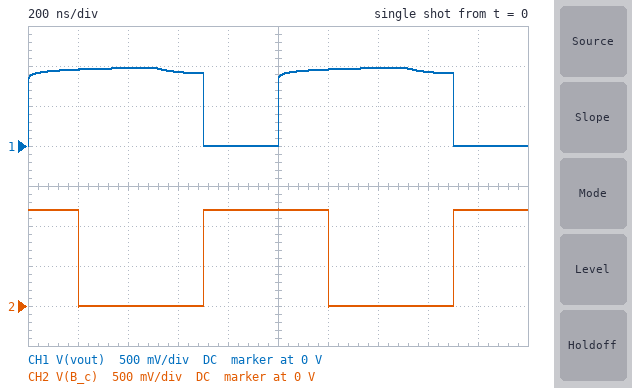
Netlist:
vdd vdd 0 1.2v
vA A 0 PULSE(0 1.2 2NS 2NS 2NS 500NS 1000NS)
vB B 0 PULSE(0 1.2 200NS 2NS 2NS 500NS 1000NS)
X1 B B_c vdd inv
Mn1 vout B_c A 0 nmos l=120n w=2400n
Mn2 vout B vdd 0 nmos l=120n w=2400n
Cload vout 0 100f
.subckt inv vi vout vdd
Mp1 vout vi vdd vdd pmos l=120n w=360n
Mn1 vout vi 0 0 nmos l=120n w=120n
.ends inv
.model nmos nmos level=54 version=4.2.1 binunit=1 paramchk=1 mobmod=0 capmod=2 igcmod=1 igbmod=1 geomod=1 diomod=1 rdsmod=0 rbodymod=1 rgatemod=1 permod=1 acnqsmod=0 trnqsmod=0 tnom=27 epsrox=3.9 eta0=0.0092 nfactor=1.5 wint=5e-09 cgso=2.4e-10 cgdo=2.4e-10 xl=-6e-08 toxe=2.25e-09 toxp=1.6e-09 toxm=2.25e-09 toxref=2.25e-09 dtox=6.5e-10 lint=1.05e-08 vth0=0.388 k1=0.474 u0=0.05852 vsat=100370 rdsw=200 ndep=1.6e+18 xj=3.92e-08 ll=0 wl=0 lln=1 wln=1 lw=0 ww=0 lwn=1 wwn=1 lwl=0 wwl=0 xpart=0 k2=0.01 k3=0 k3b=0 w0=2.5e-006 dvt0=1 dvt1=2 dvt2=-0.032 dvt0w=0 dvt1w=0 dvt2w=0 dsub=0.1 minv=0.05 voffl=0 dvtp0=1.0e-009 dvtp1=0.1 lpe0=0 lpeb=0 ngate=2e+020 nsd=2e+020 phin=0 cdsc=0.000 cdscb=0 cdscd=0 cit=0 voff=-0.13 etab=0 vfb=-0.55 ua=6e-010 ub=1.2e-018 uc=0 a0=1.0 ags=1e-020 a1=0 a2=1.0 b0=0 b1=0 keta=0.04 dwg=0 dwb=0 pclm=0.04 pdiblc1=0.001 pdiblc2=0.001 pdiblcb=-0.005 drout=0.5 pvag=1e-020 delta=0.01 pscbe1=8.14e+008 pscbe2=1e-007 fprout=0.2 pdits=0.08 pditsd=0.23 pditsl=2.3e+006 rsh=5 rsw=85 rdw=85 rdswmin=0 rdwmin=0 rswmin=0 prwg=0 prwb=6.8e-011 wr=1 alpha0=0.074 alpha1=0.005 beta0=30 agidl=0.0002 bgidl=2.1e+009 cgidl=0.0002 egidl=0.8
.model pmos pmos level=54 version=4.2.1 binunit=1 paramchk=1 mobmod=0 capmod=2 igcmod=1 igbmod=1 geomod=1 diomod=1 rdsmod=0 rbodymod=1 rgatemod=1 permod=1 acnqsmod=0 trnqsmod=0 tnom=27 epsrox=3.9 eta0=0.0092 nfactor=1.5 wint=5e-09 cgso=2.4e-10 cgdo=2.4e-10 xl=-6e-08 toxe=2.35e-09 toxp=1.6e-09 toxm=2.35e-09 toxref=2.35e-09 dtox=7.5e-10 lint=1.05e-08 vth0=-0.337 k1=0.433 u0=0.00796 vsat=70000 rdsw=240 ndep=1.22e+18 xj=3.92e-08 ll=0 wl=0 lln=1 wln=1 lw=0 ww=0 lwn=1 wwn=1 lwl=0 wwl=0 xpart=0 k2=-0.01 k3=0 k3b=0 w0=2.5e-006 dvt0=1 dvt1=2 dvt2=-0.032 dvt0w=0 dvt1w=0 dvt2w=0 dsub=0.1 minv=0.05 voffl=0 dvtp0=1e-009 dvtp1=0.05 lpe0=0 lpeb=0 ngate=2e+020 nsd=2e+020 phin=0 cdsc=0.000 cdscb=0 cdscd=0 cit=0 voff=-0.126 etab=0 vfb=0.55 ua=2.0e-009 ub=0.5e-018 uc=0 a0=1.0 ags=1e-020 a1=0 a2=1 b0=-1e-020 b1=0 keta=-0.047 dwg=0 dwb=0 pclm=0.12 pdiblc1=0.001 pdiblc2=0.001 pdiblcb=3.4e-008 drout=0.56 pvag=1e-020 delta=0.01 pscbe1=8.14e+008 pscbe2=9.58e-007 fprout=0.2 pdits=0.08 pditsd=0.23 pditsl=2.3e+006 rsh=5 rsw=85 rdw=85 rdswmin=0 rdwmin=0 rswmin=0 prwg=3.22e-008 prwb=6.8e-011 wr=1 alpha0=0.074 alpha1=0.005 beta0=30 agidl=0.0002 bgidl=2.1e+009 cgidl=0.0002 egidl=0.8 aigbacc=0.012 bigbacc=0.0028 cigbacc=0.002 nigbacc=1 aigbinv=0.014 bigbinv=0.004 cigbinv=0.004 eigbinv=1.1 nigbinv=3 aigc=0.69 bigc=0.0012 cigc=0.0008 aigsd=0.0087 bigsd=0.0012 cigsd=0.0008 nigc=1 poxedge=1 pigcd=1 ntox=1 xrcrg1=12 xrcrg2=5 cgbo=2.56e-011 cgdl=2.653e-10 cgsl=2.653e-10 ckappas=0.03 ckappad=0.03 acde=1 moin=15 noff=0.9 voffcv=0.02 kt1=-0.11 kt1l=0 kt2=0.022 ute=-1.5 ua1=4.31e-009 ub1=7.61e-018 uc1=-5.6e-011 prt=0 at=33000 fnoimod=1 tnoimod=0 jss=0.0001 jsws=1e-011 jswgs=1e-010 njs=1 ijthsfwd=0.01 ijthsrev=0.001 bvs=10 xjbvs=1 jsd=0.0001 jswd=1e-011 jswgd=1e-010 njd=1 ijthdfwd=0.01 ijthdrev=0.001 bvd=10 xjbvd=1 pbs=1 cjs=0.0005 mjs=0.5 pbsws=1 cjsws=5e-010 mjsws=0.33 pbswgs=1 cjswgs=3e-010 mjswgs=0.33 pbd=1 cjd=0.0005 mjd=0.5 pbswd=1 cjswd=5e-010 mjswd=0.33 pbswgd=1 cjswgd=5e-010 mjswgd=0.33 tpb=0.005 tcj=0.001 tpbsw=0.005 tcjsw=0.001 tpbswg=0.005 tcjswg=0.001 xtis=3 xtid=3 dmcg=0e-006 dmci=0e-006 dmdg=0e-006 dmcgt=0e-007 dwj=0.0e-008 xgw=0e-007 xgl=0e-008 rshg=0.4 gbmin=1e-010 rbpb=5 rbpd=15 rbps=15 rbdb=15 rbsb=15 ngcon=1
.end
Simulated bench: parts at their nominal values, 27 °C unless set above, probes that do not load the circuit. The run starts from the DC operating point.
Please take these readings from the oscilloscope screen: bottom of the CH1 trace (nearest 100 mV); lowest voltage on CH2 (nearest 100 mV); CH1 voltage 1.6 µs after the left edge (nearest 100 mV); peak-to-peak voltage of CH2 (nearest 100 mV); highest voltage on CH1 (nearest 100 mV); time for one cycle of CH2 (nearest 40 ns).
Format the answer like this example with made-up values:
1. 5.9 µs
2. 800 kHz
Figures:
1. 0 V
2. 0 V
3. 900 mV
4. 1.2 V
5. 1.0 V
6. 1.00 µs
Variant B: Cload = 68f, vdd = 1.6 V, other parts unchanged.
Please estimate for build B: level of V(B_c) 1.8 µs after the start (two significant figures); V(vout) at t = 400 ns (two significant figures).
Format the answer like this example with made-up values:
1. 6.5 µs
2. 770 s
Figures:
1. 1.6 V
2. 1.2 V
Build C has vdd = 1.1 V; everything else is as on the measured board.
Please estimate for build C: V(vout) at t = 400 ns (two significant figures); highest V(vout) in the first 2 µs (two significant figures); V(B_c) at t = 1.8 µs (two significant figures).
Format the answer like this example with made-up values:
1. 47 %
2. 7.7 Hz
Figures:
1. 950 mV
2. 960 mV
3. 1.1 V
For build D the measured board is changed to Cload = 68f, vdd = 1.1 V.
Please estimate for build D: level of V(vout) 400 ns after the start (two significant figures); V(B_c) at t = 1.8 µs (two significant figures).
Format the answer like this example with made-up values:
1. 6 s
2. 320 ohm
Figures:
1. 960 mV
2. 1.1 V
